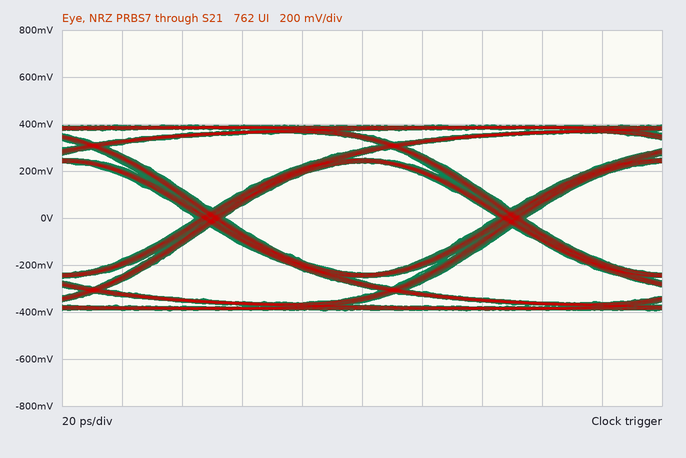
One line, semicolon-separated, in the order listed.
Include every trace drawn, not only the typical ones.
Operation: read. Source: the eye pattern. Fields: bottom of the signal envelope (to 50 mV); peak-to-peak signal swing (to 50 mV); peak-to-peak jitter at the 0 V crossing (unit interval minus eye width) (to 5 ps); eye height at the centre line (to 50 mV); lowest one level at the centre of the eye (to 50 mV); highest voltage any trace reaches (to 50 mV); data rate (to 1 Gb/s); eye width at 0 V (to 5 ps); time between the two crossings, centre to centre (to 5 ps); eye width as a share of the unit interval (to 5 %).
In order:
-400 mV; 800 mV; 10 ps; 450 mV; 250 mV; 400 mV; 10 Gb/s; 90 ps; 100 ps; 90 %
